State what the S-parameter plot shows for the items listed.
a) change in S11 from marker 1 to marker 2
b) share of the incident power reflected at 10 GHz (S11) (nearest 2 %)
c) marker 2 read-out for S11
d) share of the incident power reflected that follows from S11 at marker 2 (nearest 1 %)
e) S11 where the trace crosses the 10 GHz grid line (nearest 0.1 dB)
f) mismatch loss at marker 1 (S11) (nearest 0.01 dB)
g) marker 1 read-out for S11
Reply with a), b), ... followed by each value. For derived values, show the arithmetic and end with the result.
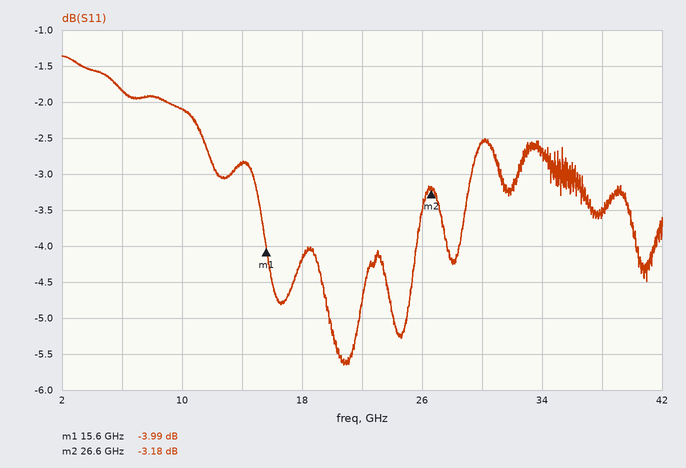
a) -3.18 − (-3.99) = 0.81 dB
b) 10^(-2.1/10) ≈ 62 %
c) -3.18 dB
d) 10^(-3.18/10) ≈ 48 %
e) -2.1 dB
f) −10 log10(1 − 10^(-3.99/10)) ≈ 2.21 dB
g) -3.99 dB
